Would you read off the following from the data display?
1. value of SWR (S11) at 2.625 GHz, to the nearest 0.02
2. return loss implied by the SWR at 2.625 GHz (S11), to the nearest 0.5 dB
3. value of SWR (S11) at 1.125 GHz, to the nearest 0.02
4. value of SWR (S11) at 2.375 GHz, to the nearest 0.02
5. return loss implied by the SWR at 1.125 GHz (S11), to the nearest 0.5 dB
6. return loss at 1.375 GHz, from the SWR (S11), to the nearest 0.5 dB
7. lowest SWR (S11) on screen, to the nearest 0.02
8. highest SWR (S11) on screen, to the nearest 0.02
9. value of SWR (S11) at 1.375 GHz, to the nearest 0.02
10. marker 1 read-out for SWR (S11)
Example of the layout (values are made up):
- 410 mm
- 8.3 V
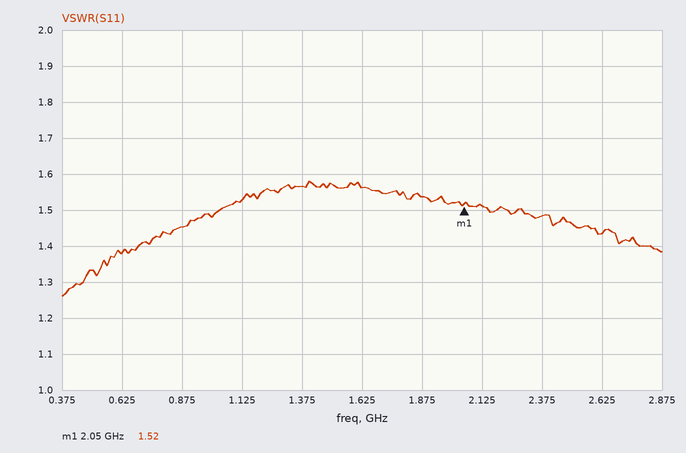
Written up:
- 1.44
- 15.0 dB
- 1.52
- 1.48
- 13.5 dB
- 13.0 dB
- 1.26
- 1.58
- 1.56
- 1.52
